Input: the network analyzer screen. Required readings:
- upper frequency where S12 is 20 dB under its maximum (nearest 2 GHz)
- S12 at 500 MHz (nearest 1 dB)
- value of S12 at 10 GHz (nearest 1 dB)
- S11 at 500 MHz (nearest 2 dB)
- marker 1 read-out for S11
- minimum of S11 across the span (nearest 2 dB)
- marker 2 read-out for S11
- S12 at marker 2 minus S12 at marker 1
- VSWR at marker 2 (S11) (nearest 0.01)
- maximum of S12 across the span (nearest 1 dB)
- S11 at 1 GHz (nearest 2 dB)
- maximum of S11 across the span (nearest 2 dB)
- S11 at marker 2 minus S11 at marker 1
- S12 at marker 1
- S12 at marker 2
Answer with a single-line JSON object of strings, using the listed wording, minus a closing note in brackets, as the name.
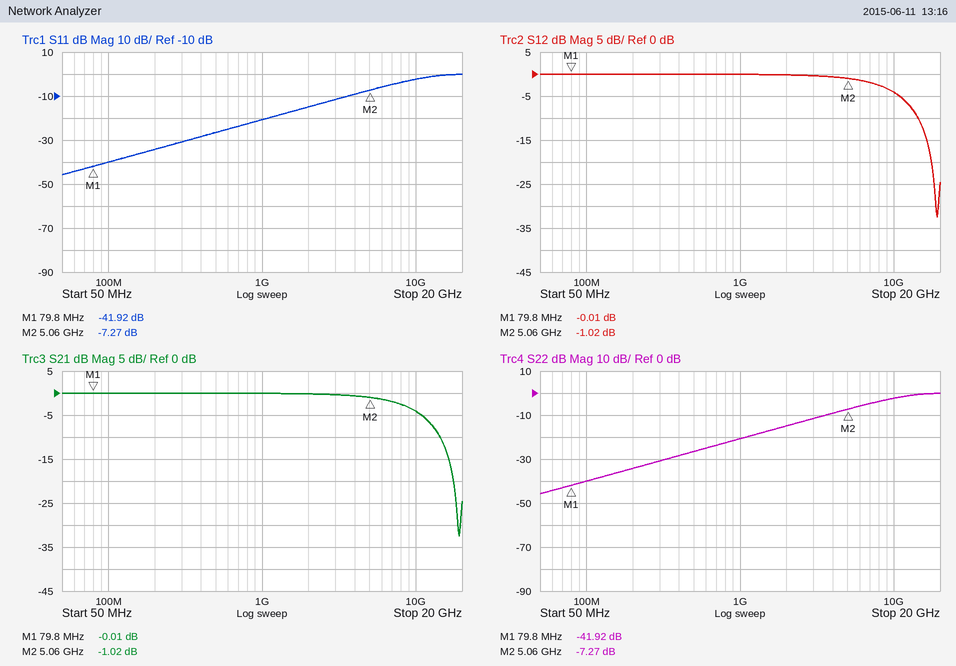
{"upper frequency where S12 is 20 dB under its maximum": "18 GHz", "S12 at 500 MHz": "0 dB", "value of S12 at 10 GHz": "-4 dB", "S11 at 500 MHz": "-26 dB", "marker 1 read-out for S11": "-41.92 dB", "minimum of S11 across the span": "-46 dB", "marker 2 read-out for S11": "-7.27 dB", "S12 at marker 2 minus S12 at marker 1": "-1.01 dB", "VSWR at marker 2 (S11)": "2.53", "maximum of S12 across the span": "0 dB", "S11 at 1 GHz": "-20 dB", "maximum of S11 across the span": "0 dB", "S11 at marker 2 minus S11 at marker 1": "34.65 dB", "S12 at marker 1": "-0.01 dB", "S12 at marker 2": "-1.02 dB"}
